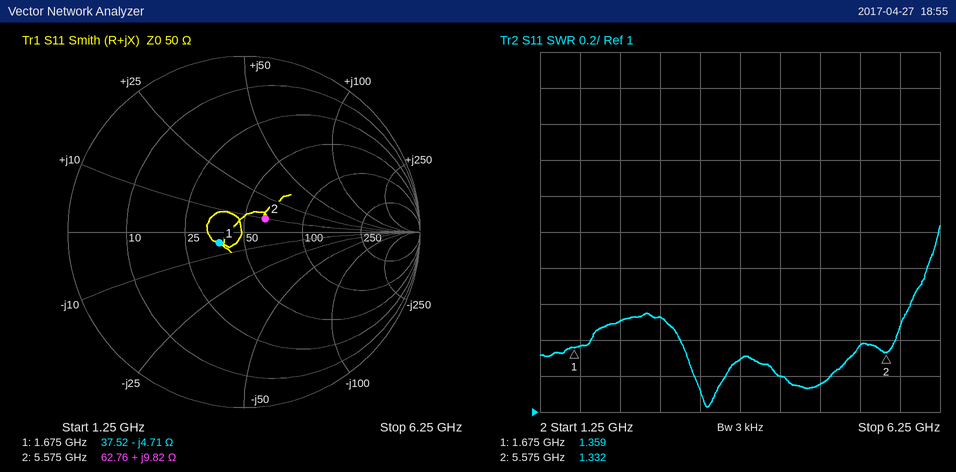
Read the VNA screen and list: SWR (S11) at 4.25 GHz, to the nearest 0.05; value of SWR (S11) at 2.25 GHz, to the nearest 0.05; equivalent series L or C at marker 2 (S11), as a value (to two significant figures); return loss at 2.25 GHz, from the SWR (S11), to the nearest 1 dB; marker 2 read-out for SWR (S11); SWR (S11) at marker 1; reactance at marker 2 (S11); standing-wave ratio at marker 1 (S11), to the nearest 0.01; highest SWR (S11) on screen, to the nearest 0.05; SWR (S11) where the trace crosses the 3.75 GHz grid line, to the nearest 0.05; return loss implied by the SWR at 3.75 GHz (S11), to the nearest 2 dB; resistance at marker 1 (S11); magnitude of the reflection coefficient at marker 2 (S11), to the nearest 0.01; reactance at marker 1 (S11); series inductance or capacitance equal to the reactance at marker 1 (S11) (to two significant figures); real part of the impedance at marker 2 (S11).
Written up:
1.20
1.50
280 pH
14 dB
1.332
1.359
+9.82 Ω
1.36
2.05
1.30
18 dB
37.52 Ω
0.14
-4.71 Ω
20 pF
62.76 Ω
